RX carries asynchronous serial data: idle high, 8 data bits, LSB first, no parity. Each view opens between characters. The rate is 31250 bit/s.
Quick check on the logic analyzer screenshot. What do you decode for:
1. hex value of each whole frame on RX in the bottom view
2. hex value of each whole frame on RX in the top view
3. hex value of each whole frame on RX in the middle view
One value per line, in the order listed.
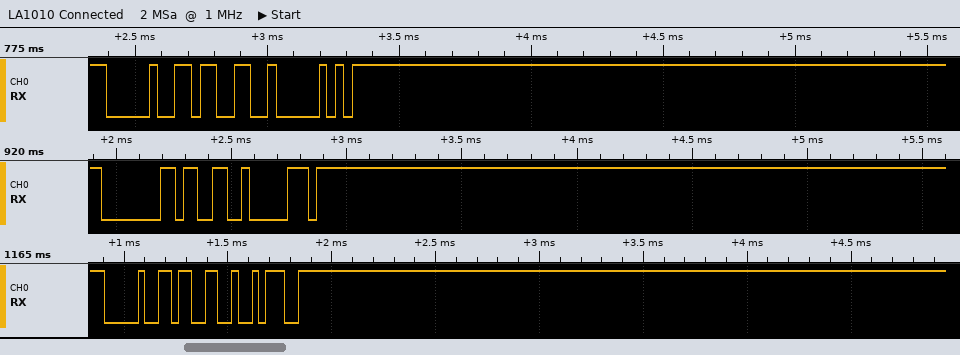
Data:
90, 33, 3A
90, 33, 50
80, 33, 70
